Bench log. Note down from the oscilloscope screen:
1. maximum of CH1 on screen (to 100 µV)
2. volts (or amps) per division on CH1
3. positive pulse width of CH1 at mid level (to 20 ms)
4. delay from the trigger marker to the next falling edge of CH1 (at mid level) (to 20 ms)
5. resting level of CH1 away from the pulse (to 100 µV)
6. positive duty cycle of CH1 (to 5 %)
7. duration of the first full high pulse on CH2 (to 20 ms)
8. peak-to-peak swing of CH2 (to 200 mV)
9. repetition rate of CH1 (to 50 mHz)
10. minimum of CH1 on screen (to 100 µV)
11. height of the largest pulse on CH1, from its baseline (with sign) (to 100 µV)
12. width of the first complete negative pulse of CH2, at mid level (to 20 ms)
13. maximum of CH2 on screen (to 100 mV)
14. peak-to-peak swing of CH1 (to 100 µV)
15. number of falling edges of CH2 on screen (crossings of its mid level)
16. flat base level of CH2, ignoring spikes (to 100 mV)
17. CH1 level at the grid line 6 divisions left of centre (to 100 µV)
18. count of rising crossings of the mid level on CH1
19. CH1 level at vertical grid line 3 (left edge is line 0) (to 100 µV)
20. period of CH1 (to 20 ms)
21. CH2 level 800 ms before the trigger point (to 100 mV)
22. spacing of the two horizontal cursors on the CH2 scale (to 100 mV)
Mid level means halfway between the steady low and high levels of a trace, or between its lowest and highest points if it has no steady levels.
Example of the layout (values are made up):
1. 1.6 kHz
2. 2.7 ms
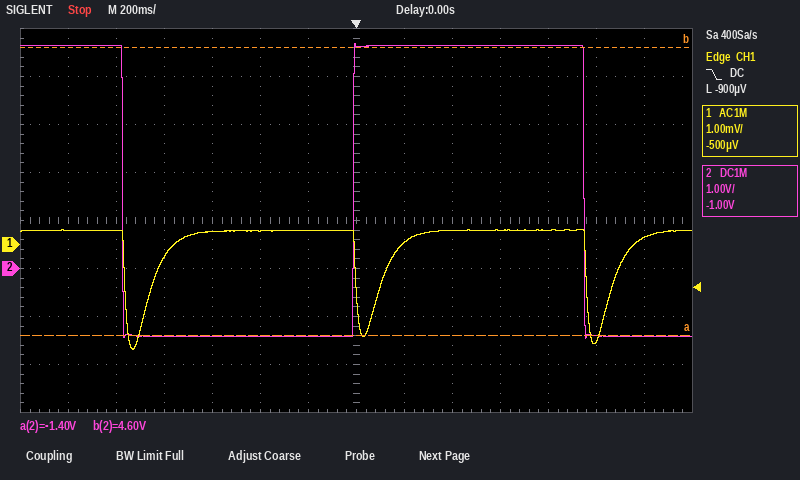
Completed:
1. 300 µV
2. 1 mV
3. 860 ms
4. 960 ms
5. 300 µV
6. 90 %
7. 960 ms
8. 6.2 V
9. 1.05 Hz
10. -2.2 mV
11. -2.5 mV
12. 960 ms
13. 4.7 V
14. 2.5 mV
15. 2
16. -1.4 V
17. 300 µV
18. 3
19. -300 µV
20. 960 ms
21. -1.4 V
22. 6.0 V
